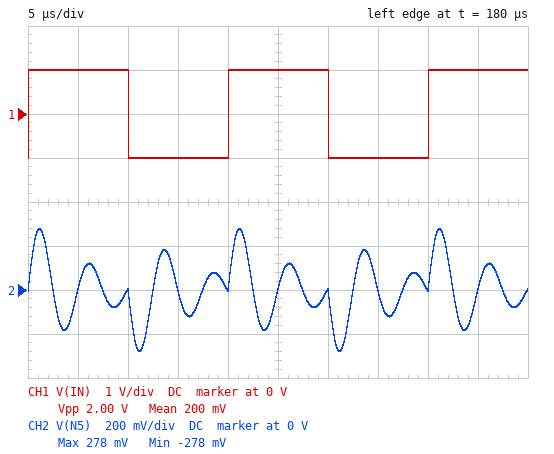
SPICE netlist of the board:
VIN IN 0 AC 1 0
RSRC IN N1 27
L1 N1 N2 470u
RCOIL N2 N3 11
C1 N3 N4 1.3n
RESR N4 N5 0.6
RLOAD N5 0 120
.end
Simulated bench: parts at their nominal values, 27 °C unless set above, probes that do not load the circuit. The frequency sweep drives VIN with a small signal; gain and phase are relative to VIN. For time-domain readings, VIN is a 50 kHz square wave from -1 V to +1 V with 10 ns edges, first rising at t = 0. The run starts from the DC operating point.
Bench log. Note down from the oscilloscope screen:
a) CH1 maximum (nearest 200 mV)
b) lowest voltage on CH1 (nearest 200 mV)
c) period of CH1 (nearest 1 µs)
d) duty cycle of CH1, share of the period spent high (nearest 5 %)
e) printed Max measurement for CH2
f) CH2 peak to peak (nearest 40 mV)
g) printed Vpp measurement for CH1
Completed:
1.0 V
-1.0 V
20 µs
50 %
278 mV
560 mV
2.00 V
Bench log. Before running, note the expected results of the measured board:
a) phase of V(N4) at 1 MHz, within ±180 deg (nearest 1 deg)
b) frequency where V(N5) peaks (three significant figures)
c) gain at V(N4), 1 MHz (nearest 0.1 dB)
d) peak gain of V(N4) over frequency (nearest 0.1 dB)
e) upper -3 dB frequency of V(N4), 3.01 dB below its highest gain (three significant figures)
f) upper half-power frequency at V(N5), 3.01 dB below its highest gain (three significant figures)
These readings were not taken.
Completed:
-87 deg
204 kHz
-27.4 dB
-2.4 dB
232 kHz
232 kHz
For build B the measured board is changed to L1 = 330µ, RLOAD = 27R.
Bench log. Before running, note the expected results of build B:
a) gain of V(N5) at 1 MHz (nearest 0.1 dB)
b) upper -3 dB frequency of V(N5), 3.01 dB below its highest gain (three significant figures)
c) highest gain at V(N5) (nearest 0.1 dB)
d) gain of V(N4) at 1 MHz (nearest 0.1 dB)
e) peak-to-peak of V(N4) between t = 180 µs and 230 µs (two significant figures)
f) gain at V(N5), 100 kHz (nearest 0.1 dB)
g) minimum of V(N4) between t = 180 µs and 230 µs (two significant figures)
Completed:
-37.2 dB
259 kHz
-7.7 dB
-37.0 dB
280 mV
-31.5 dB
-140 mV
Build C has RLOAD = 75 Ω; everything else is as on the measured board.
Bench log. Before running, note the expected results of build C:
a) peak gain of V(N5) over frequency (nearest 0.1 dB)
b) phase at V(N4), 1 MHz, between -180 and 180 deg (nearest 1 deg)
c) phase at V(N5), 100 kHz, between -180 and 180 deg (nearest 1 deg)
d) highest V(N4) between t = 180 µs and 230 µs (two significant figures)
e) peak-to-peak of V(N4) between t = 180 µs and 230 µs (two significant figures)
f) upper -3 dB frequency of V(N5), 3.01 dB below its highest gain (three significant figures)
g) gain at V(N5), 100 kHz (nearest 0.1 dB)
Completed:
-3.6 dB
-88 deg
83 deg
170 mV
340 mV
224 kHz
-21.9 dB
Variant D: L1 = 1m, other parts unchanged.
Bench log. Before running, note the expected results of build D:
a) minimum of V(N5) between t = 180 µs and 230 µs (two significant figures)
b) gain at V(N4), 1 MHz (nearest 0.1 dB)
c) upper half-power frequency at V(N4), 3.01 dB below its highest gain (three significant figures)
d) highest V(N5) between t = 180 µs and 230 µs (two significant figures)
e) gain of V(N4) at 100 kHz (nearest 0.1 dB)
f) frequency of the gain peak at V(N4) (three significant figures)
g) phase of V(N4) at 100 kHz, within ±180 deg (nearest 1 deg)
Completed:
-320 mV
-34.2 dB
153 kHz
320 mV
-14.2 dB
140 kHz
75 deg
